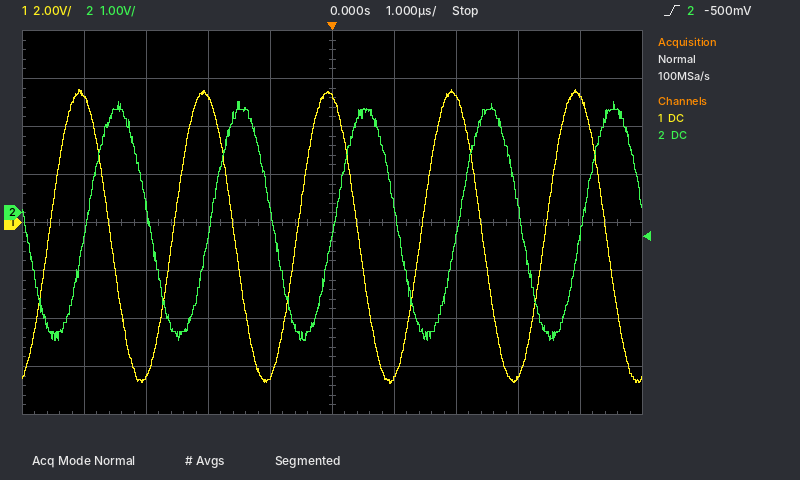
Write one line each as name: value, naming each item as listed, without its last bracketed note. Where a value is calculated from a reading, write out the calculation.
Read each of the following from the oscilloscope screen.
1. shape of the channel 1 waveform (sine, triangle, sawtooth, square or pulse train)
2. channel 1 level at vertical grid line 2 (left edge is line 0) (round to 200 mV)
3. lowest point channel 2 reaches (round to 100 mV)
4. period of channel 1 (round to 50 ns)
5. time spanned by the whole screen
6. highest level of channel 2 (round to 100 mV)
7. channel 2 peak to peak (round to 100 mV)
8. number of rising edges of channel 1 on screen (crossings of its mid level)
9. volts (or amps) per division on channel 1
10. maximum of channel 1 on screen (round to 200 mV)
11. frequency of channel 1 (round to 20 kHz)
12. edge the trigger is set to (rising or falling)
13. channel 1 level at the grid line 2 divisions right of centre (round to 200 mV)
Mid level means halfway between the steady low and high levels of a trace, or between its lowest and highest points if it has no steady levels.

shape of the channel 1 waveform: sine
channel 1 level at vertical grid line 2 (left edge is line 0): -6.4 V
lowest point channel 2 reaches: -2.7 V
period of channel 1: 2.00 µs
time spanned by the whole screen: 10 µs
highest level of channel 2: 2.3 V
channel 2 peak to peak: 2.3 V − (-2.7 V) = 5.0 V
number of rising edges of channel 1 on screen: 5
volts (or amps) per division on channel 1: 2 V
maximum of channel 1 on screen: 5.6 V
frequency of channel 1: 1 / 2.00 µs ≈ 500 kHz
edge the trigger is set to: rising
channel 1 level at the grid line 2 divisions right of centre: 5.2 V
